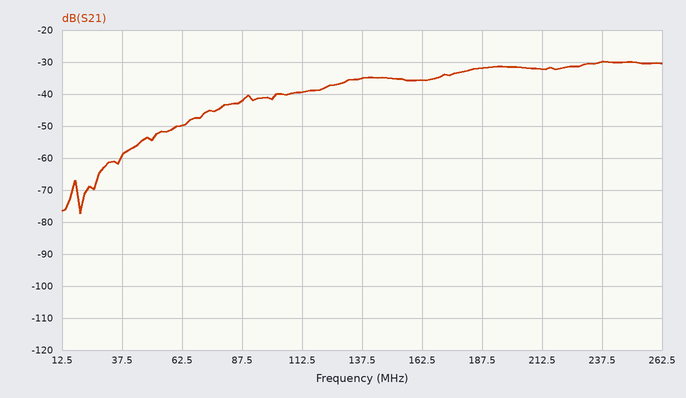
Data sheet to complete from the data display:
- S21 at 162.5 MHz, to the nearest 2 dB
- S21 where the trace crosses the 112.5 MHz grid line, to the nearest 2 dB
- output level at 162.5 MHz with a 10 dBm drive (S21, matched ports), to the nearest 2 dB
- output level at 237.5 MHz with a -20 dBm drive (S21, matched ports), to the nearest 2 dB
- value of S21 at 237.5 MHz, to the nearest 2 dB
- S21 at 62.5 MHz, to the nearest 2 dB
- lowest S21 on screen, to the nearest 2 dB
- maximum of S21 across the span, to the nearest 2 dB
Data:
-36 dB
-40 dB
-26 dBm
-50 dBm
-30 dB
-50 dB
-78 dB
-30 dB
